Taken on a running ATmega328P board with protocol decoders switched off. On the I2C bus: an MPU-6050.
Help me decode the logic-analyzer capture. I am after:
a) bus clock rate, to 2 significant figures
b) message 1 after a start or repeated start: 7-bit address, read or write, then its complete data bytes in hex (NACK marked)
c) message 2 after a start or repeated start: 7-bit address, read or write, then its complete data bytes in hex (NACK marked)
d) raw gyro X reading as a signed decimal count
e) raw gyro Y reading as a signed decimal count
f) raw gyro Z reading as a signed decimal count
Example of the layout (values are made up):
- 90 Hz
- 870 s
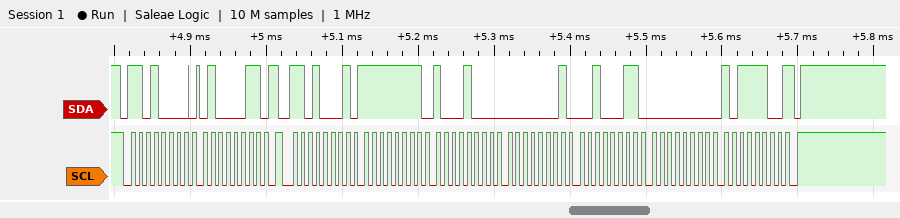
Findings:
- 100 kHz
- 0x68 write: 43
- 0x68 read: FF 88 01 23 00 BC NACK
- -120
- 291
- 188
